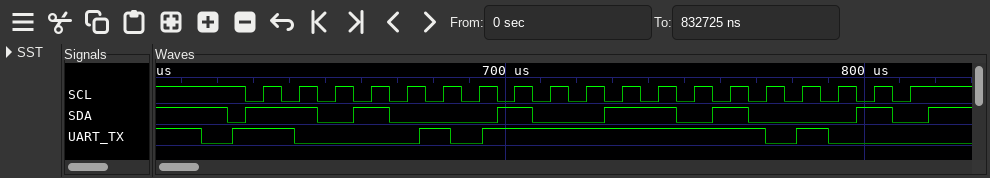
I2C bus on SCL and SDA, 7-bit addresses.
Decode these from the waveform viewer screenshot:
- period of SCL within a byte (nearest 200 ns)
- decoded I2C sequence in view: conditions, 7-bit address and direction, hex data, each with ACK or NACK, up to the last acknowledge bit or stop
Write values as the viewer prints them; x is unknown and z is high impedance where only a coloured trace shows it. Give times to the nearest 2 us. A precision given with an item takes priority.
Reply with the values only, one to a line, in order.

10000 ns
start, address 68 read ACK, 68 NACK, stop
